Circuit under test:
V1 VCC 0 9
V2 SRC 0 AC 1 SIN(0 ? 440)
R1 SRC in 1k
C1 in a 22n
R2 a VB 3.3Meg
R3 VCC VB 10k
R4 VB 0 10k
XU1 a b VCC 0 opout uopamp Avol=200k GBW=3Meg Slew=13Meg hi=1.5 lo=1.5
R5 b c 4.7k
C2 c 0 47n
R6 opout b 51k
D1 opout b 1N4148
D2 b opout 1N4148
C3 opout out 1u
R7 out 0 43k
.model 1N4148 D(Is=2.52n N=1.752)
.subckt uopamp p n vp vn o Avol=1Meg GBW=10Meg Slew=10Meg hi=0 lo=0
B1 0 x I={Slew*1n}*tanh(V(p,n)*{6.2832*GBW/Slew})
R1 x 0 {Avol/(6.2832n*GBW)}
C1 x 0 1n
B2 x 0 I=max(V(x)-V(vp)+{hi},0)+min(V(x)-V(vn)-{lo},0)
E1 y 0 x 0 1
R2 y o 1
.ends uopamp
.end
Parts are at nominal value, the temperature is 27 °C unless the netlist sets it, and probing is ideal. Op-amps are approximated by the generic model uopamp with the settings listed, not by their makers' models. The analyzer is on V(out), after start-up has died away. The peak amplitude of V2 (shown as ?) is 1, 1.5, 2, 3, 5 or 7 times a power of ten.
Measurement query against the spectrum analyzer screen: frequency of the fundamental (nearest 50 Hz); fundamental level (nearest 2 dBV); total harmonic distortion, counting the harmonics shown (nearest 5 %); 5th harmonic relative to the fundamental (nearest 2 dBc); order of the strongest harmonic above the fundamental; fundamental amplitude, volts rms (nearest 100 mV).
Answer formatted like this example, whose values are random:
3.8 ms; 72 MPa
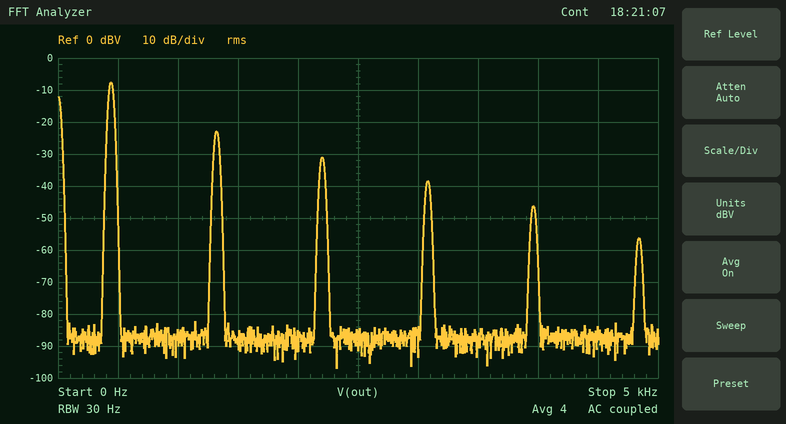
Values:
450 Hz; -8 dBV; 20 %; -24 dBc; 3; 400 mV
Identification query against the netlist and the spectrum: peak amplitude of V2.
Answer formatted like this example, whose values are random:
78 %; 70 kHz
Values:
200 mV
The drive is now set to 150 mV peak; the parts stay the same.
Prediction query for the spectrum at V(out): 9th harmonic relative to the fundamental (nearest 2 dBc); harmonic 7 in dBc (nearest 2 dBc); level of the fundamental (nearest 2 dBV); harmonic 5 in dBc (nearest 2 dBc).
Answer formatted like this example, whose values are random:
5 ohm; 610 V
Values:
-52 dBc; -36 dBc; -8 dBV; -26 dBc
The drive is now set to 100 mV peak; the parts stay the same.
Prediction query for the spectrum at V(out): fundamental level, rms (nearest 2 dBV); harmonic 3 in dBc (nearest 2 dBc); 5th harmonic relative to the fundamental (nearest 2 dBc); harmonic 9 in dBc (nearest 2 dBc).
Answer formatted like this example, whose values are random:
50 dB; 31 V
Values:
-10 dBV; -18 dBc; -34 dBc; -50 dBc
